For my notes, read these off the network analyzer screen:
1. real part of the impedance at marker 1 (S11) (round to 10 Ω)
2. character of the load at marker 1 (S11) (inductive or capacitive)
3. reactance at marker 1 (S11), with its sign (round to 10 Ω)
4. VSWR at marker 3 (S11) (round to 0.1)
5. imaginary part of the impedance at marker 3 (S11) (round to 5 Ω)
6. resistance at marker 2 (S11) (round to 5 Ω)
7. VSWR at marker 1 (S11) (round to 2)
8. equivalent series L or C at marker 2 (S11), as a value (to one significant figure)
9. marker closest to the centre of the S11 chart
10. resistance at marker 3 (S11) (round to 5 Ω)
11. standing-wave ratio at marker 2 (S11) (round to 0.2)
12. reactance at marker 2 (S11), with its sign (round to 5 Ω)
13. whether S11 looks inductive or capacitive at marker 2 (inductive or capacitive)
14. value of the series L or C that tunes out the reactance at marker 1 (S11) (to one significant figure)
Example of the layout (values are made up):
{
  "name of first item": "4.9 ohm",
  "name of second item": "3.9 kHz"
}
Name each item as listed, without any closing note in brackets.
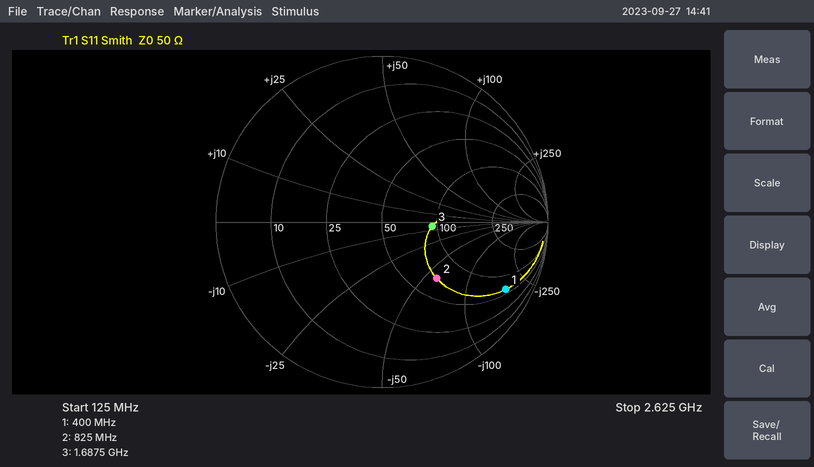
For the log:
{
  "real part of the impedance at marker 1 (S11)": "60 Ω",
  "character of the load at marker 1 (S11)": "capacitive",
  "reactance at marker 1 (S11), with its sign": "-180 Ω",
  "VSWR at marker 3 (S11)": "1.9",
  "imaginary part of the impedance at marker 3 (S11)": "-5 Ω",
  "resistance at marker 2 (S11)": "70 Ω",
  "VSWR at marker 1 (S11)": "12",
  "equivalent series L or C at marker 2 (S11), as a value": "3 pF",
  "marker closest to the centre of the S11 chart": "marker 3",
  "resistance at marker 3 (S11)": "95 Ω",
  "standing-wave ratio at marker 2 (S11)": "2.8",
  "reactance at marker 2 (S11), with its sign": "-60 Ω",
  "whether S11 looks inductive or capacitive at marker 2": "capacitive",
  "value of the series L or C that tunes out the reactance at marker 1 (S11)": "70 nH"
}
